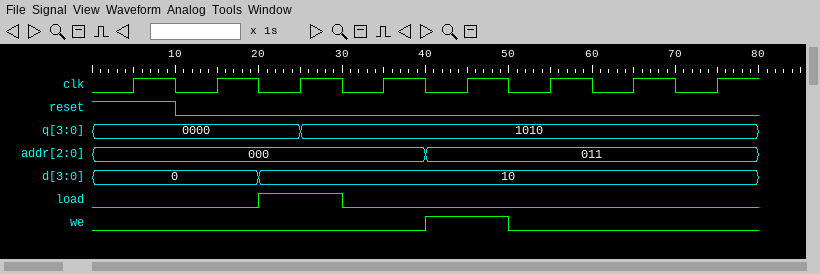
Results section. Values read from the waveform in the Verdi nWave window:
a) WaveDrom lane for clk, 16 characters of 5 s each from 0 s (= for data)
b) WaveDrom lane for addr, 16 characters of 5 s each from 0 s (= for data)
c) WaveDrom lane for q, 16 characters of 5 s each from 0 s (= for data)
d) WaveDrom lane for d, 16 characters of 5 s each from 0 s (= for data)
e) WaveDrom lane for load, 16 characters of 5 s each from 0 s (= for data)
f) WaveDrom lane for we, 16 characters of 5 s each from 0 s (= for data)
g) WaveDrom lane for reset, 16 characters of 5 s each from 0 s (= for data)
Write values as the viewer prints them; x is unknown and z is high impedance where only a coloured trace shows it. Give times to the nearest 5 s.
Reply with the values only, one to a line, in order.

{name: 'clk', wave: '0101010101010101'}
{name: 'addr', wave: '=.......=.......', data: '000 011'}
{name: 'q', wave: '=....=..........', data: '0000 1010'}
{name: 'd', wave: '=...=...........', data: '0 10'}
{name: 'load', wave: '0...1.0.........'}
{name: 'we', wave: '0.......1.0.....'}
{name: 'reset', wave: '1.0.............'}
